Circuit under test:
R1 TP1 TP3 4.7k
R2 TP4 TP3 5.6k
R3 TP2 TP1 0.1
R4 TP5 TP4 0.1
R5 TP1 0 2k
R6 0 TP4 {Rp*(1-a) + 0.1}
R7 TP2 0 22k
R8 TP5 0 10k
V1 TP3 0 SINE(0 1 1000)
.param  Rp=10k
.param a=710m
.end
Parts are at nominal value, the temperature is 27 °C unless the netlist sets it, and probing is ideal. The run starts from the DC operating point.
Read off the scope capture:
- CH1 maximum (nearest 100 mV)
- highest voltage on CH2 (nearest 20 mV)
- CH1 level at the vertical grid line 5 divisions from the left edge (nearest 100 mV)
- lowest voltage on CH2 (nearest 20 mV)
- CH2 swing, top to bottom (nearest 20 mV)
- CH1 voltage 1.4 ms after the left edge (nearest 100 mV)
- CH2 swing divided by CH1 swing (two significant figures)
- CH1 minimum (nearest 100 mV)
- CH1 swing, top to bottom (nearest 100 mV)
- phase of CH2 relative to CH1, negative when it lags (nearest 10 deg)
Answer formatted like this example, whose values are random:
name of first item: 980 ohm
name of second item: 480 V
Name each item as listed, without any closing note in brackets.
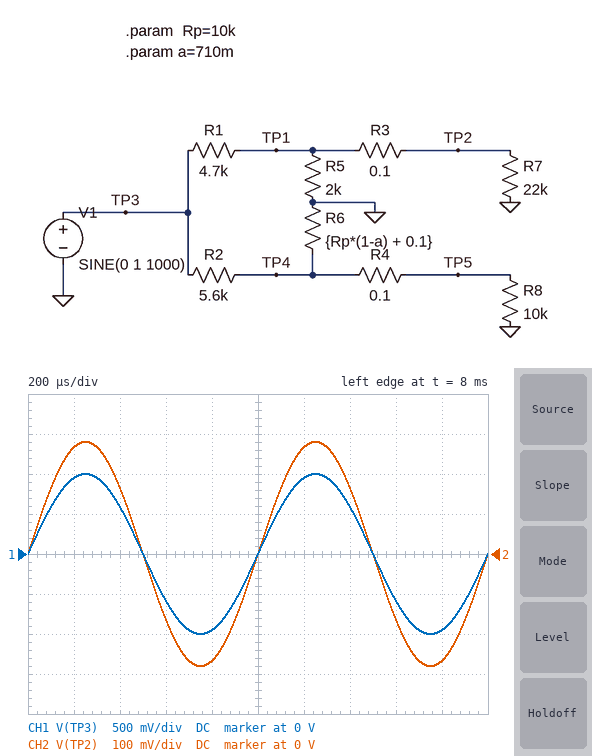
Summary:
CH1 maximum: 1.0 V
highest voltage on CH2: 280 mV
CH1 level at the vertical grid line 5 divisions from the left edge: 0 V
lowest voltage on CH2: -280 mV
CH2 swing, top to bottom: 560 mV
CH1 voltage 1.4 ms after the left edge: 600 mV
CH2 swing divided by CH1 swing: 0.28
CH1 minimum: -1.0 V
CH1 swing, top to bottom: 2.0 V
phase of CH2 relative to CH1, negative when it lags: 0 deg
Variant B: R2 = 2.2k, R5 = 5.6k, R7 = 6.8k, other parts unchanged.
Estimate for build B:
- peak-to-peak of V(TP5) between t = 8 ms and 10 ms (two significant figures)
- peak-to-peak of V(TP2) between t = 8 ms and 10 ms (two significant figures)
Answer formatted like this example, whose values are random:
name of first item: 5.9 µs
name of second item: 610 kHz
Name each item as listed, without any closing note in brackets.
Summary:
peak-to-peak of V(TP5) between t = 8 ms and 10 ms: 1.0 V
peak-to-peak of V(TP2) between t = 8 ms and 10 ms: 790 mV
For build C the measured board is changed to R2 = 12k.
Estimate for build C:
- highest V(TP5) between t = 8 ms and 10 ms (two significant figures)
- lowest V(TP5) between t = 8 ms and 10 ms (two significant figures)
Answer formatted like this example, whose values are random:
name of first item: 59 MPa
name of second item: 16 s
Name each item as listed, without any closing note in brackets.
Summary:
highest V(TP5) between t = 8 ms and 10 ms: 160 mV
lowest V(TP5) between t = 8 ms and 10 ms: -160 mV
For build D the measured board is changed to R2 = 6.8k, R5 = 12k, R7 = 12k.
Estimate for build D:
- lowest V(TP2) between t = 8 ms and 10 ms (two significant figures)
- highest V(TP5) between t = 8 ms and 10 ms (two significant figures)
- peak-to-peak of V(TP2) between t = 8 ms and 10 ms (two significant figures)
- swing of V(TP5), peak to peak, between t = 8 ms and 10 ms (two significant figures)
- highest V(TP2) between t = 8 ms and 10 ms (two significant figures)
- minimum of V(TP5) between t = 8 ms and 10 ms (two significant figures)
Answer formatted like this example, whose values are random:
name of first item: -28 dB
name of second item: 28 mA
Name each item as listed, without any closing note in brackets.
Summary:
lowest V(TP2) between t = 8 ms and 10 ms: -560 mV
highest V(TP5) between t = 8 ms and 10 ms: 250 mV
peak-to-peak of V(TP2) between t = 8 ms and 10 ms: 1.1 V
swing of V(TP5), peak to peak, between t = 8 ms and 10 ms: 500 mV
highest V(TP2) between t = 8 ms and 10 ms: 560 mV
minimum of V(TP5) between t = 8 ms and 10 ms: -250 mV
